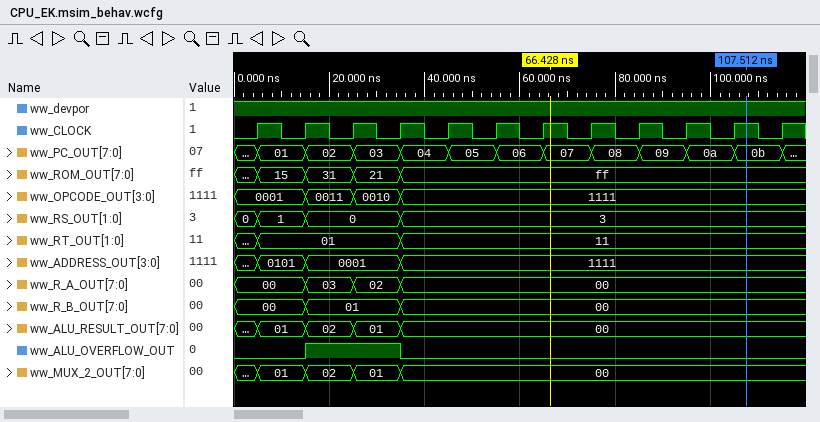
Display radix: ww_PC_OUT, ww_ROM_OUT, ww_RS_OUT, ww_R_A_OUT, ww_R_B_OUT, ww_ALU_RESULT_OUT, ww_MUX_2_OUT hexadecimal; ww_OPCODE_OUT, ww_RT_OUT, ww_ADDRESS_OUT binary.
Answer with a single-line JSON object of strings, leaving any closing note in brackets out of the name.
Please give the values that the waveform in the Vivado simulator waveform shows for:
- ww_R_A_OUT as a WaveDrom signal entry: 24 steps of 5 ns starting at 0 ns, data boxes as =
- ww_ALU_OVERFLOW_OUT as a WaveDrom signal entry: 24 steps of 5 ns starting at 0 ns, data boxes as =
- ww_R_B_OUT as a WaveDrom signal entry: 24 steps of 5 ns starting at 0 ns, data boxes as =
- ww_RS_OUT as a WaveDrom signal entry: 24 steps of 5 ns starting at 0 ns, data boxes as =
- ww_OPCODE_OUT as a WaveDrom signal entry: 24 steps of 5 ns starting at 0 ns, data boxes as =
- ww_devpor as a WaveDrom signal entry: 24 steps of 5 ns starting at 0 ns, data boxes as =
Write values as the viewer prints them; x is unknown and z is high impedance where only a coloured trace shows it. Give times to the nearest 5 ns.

{"ww_R_A_OUT as a WaveDrom signal entry: 24 steps of 5 ns starting at 0 ns, data boxes as =": "{name: 'ww_R_A_OUT', wave: '=..=.=.=................', data: '00 03 02 00'}", "ww_ALU_OVERFLOW_OUT as a WaveDrom signal entry: 24 steps of 5 ns starting at 0 ns, data boxes as =": "{name: 'ww_ALU_OVERFLOW_OUT', wave: '0..1...0................'}", "ww_R_B_OUT as a WaveDrom signal entry: 24 steps of 5 ns starting at 0 ns, data boxes as =": "{name: 'ww_R_B_OUT', wave: '=..=...=................', data: '00 01 00'}", "ww_RS_OUT as a WaveDrom signal entry: 24 steps of 5 ns starting at 0 ns, data boxes as =": "{name: 'ww_RS_OUT', wave: '==.=...=................', data: '0 1 0 3'}", "ww_OPCODE_OUT as a WaveDrom signal entry: 24 steps of 5 ns starting at 0 ns, data boxes as =": "{name: 'ww_OPCODE_OUT', wave: '=..=.=.=................', data: '0001 0011 0010 1111'}", "ww_devpor as a WaveDrom signal entry: 24 steps of 5 ns starting at 0 ns, data boxes as =": "{name: 'ww_devpor', wave: '1.......................'}"}
